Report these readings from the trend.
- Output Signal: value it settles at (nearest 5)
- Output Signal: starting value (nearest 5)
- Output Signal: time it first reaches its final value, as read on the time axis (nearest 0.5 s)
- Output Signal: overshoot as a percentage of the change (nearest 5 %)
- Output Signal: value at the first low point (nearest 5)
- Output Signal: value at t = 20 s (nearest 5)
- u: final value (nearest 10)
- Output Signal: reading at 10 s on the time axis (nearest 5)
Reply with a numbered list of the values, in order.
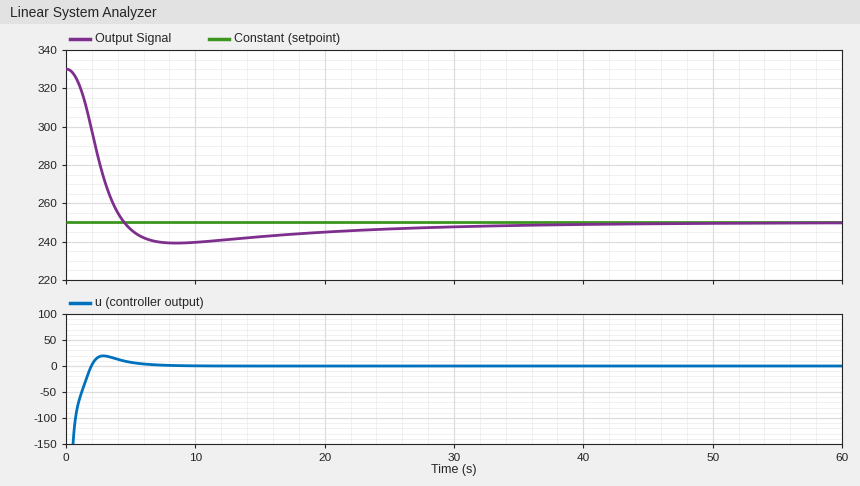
1. 250
2. 330
3. 4.5 s
4. 15 %
5. 240
6. 245
7. 0
8. 240
